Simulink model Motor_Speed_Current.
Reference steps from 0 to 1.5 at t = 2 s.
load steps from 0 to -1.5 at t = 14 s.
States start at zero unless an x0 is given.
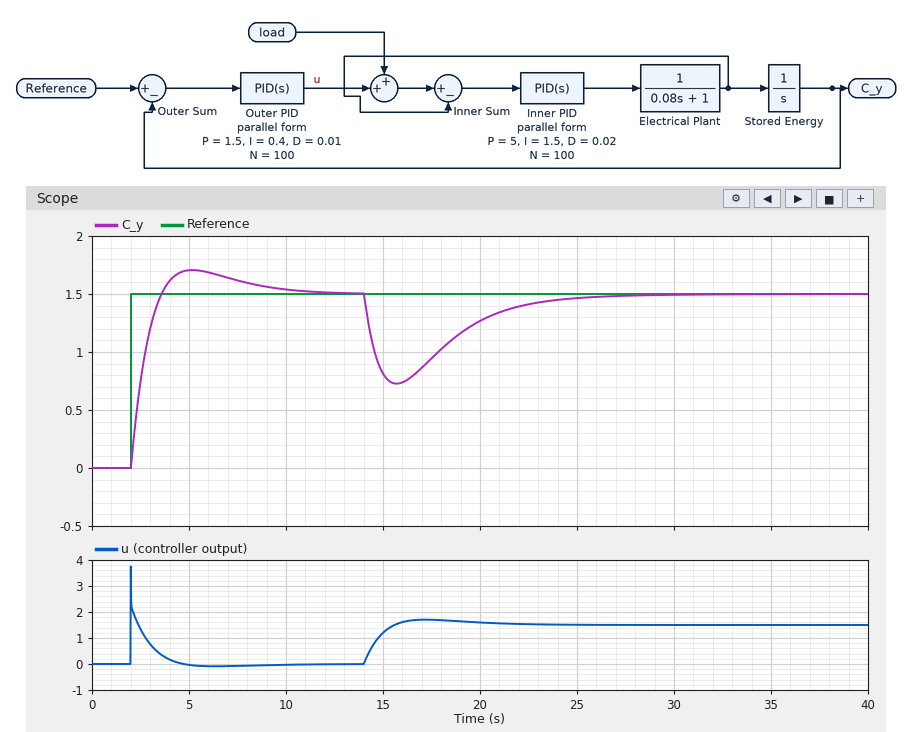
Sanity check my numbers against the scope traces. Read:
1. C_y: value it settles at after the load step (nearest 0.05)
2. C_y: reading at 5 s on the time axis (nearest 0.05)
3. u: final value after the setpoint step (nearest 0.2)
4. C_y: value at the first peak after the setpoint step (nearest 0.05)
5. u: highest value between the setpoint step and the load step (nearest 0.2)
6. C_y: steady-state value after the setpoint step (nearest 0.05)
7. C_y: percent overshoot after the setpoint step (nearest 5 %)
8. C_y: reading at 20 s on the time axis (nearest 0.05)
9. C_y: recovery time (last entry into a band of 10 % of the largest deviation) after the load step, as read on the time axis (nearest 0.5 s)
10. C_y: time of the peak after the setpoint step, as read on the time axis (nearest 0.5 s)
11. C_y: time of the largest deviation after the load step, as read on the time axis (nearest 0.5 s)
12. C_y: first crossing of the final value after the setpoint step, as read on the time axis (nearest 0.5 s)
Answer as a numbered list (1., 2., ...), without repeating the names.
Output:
1. 1.50
2. 1.70
3. 0.0
4. 1.70
5. 3.8
6. 1.50
7. 15 %
8. 1.25
9. 23.0 s
10. 5.0 s
11. 15.5 s
12. 3.5 s
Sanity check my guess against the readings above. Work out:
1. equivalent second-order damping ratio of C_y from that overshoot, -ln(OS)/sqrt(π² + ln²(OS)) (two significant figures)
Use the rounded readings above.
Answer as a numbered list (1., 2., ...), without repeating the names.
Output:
1. 0.52
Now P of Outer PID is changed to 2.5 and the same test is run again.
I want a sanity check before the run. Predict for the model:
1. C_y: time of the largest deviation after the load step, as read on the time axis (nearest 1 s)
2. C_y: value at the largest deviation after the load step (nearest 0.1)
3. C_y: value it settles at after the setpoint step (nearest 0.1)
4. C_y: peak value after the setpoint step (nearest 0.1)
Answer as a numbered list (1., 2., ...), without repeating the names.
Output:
1. 15 s
2. 1.0
3. 1.5
4. 1.6
